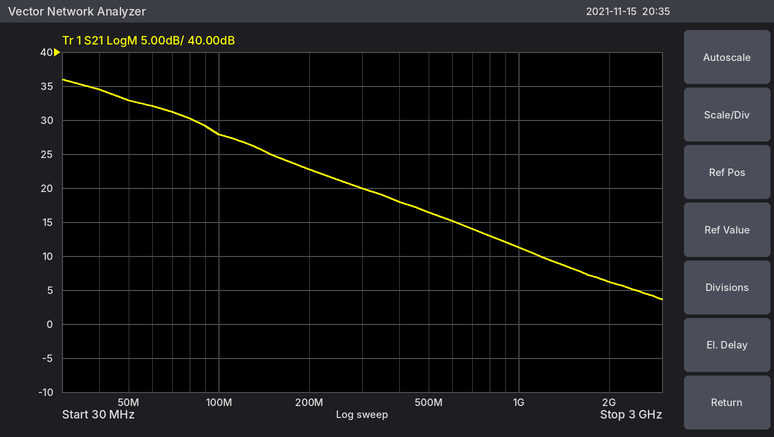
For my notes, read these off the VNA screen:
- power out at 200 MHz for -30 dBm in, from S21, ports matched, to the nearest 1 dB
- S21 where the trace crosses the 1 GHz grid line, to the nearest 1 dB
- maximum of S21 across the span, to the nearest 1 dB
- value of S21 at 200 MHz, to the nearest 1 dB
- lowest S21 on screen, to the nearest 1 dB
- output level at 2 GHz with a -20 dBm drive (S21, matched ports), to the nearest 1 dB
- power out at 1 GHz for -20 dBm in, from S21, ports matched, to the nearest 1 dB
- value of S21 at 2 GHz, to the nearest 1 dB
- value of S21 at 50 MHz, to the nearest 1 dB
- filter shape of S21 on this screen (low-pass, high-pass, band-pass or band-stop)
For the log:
-7 dBm
11 dB
36 dB
23 dB
4 dB
-14 dBm
-9 dBm
6 dB
33 dB
low-pass
